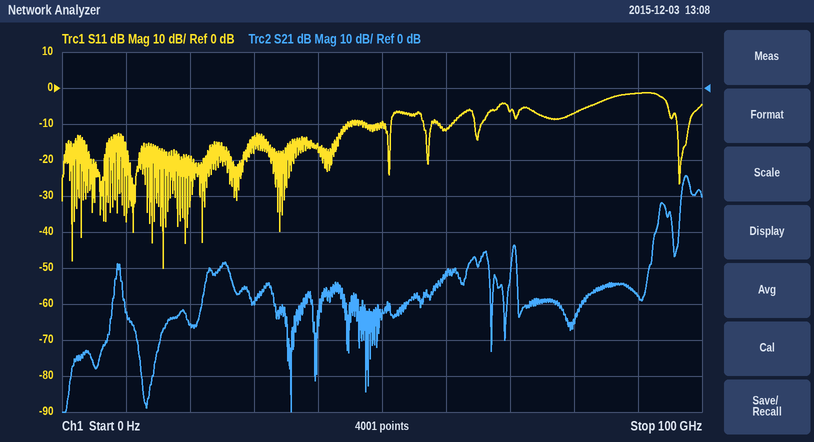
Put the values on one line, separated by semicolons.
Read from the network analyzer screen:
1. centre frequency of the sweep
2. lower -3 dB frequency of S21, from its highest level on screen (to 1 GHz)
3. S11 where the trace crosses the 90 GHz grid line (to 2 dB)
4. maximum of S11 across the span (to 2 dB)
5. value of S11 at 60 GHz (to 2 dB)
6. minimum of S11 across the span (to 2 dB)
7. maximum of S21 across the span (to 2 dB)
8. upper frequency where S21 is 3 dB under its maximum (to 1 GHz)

50 GHz; 97 GHz; -2 dB; -2 dB; -12 dB; -50 dB; -24 dB; 98 GHz
